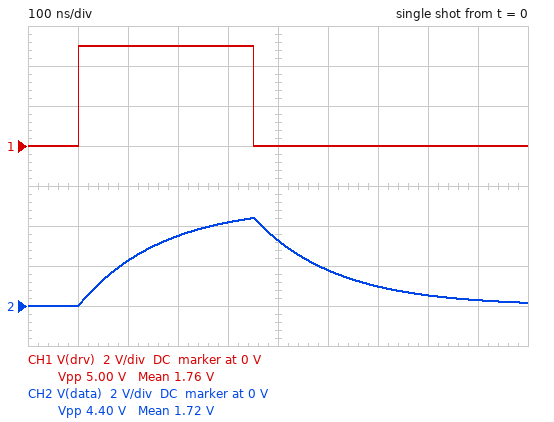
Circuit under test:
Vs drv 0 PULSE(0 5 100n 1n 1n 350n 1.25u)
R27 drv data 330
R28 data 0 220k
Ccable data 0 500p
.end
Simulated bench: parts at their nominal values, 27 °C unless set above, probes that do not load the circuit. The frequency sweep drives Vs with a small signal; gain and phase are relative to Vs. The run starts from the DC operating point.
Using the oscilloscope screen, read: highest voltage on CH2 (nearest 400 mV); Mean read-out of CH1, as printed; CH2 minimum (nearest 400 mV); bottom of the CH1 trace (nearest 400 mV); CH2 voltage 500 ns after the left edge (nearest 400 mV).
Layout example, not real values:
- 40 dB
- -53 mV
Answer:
- 4.4 V
- 1.76 V
- 0 V
- 0 V
- 3.2 V
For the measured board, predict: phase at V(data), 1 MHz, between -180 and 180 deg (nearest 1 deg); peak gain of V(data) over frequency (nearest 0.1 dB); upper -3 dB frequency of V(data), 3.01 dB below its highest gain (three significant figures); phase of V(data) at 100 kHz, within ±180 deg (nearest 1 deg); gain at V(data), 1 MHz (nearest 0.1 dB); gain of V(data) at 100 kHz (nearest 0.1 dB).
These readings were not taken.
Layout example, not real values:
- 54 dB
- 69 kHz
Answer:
- -46 deg
- 0 dB
- 966 kHz
- -6 deg
- -3.2 dB
- -0.1 dB
